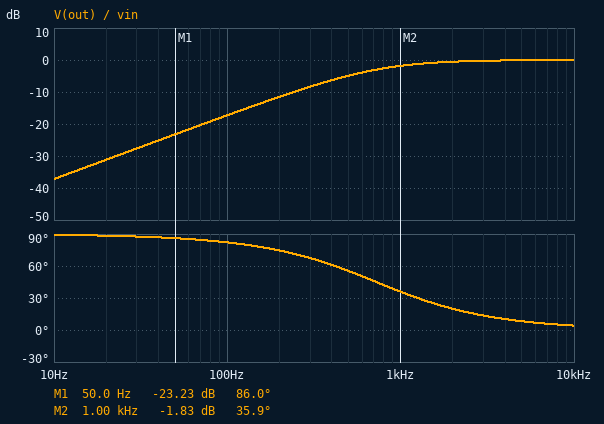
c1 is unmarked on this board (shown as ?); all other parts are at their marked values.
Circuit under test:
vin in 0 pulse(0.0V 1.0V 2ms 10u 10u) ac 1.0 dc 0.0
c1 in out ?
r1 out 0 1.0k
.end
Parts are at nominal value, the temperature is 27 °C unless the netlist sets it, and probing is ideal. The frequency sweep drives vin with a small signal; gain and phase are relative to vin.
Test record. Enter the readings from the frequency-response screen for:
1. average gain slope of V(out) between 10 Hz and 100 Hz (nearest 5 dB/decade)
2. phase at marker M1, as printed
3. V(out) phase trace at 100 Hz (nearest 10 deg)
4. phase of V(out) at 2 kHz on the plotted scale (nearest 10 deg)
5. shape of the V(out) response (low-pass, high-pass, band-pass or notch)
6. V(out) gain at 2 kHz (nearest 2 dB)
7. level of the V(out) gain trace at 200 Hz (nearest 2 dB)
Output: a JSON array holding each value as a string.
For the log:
["20 dB/decade", "86.0 deg", "80 deg", "20 deg", "high-pass", "0 dB", "-12 dB"]
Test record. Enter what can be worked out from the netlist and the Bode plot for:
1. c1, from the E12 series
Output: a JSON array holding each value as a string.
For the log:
["220 nF"]
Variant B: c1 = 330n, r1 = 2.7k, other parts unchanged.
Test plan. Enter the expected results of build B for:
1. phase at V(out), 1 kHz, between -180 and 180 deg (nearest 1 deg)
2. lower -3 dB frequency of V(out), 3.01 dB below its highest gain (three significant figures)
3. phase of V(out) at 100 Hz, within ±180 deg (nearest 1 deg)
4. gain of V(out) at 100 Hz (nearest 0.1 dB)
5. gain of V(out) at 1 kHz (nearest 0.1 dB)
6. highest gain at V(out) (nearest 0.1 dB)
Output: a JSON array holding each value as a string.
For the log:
["10 deg", "179 Hz", "61 deg", "-6.2 dB", "-0.1 dB", "0 dB"]
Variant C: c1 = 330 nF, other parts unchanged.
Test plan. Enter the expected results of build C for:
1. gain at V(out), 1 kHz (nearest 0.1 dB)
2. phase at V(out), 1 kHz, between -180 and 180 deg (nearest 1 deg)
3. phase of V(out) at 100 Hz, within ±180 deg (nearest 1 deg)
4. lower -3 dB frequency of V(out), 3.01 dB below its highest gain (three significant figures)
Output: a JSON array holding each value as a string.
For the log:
["-0.9 dB", "26 deg", "78 deg", "482 Hz"]
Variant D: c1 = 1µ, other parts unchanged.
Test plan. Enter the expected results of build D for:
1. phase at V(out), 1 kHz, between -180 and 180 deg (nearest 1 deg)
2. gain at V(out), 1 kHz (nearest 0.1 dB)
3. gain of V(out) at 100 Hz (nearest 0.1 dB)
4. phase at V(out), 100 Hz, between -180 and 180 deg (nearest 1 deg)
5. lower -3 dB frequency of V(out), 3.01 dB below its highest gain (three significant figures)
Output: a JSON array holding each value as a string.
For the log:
["9 deg", "-0.1 dB", "-5.5 dB", "58 deg", "159 Hz"]
